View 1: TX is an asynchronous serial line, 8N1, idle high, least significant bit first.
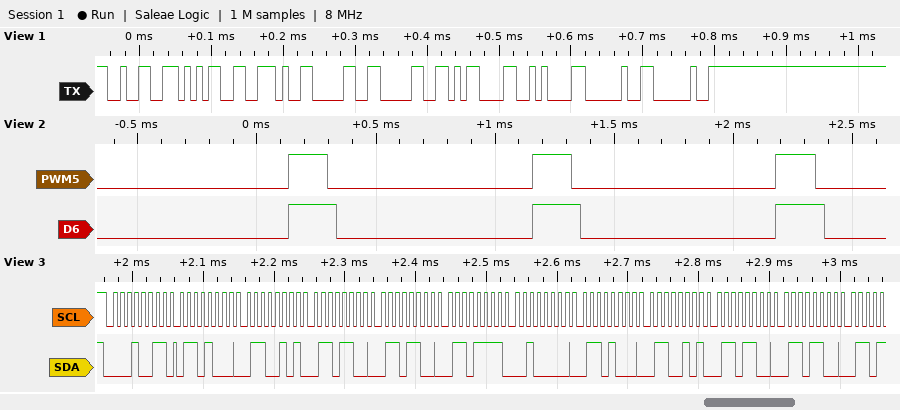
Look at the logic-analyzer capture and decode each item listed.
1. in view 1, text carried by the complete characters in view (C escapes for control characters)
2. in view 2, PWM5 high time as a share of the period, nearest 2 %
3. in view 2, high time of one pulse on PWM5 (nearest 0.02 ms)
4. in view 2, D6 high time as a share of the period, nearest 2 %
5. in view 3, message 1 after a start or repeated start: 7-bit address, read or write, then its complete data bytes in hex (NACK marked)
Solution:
"25.00\r\n  "
16 %
0.16 ms
20 %
0x09 read: 68 65 6C 6C 6F 20 68 65 6C 6C
